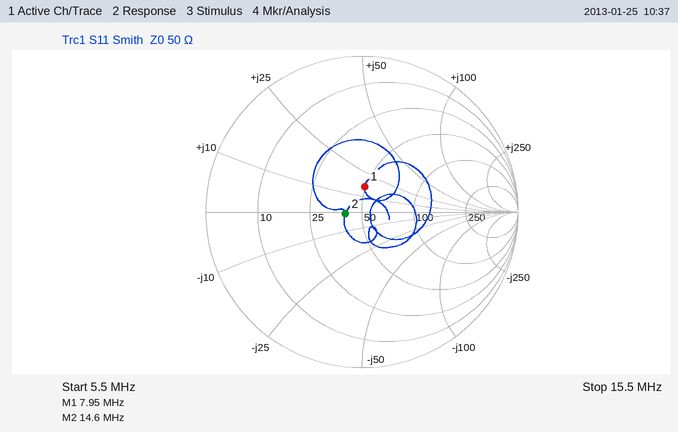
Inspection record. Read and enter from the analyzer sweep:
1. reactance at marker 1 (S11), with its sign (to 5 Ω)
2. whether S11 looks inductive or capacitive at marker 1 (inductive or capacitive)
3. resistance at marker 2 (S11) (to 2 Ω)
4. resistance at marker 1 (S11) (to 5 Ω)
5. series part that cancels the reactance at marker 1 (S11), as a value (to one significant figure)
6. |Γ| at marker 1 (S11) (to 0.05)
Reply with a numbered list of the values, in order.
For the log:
1. +15 Ω
2. inductive
3. 40 Ω
4. 50 Ω
5. 1 nF
6. 0.15
